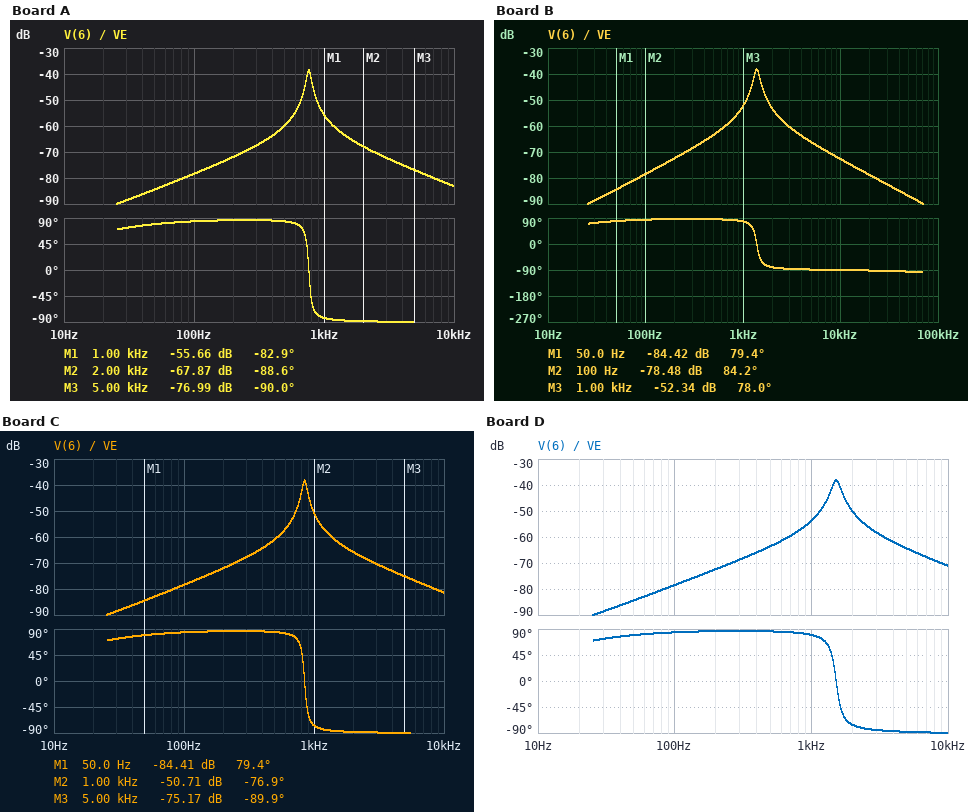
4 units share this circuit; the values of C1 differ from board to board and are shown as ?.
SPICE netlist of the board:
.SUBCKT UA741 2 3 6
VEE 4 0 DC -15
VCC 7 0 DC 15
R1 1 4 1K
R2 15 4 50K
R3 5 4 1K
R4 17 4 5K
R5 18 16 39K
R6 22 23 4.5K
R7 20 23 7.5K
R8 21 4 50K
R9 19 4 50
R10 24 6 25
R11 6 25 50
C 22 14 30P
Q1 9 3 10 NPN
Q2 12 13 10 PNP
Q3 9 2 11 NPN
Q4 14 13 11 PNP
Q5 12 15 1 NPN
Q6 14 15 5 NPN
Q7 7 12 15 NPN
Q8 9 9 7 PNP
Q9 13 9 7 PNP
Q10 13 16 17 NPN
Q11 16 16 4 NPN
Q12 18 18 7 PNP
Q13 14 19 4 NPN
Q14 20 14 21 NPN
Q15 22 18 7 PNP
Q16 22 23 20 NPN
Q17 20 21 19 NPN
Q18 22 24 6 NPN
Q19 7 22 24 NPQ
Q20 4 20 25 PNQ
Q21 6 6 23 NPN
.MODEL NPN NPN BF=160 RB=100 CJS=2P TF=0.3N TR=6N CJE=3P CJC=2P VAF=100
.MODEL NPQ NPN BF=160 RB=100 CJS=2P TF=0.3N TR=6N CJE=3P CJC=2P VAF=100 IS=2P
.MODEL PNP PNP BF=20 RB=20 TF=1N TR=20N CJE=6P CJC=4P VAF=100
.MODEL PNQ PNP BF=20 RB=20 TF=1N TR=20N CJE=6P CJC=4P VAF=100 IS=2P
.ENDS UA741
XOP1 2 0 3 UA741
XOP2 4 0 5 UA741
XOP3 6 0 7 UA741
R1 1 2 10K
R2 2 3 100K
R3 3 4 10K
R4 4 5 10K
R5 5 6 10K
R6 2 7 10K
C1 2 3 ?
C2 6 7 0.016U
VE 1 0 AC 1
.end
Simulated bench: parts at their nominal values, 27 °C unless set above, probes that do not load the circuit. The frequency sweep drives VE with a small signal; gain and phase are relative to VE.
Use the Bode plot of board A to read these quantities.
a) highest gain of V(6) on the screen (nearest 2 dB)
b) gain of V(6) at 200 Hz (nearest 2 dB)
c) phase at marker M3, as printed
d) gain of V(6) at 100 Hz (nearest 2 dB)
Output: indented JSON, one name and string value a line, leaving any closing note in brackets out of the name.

{
  "highest gain of V(6) on the screen": "-38 dB",
  "gain of V(6) at 200 Hz": "-72 dB",
  "phase at marker M3, as printed": "-90.0 deg",
  "gain of V(6) at 100 Hz": "-78 dB"
}
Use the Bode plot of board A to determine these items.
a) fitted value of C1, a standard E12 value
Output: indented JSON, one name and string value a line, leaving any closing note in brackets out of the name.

{
  "fitted value of C1, a standard E12 value": "27 nF"
}
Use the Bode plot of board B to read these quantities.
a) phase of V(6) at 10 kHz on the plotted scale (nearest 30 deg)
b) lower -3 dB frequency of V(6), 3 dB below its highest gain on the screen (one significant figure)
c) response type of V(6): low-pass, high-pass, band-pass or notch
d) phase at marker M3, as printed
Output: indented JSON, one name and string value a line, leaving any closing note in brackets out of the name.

{
  "phase of V(6) at 10 kHz on the plotted scale": "-90 deg",
  "lower -3 dB frequency of V(6), 3 dB below its highest gain on the screen": "1 kHz",
  "response type of V(6): low-pass, high-pass, band-pass or notch": "band-pass",
  "phase at marker M3, as printed": "78.0 deg"
}
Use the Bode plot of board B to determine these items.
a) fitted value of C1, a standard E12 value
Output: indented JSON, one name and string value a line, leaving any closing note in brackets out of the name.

{
  "fitted value of C1, a standard E12 value": "8.2 nF"
}
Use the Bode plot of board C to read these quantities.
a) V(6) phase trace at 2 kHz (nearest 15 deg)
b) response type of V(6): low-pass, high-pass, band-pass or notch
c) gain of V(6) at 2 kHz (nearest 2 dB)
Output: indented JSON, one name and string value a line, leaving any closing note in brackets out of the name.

{
  "V(6) phase trace at 2 kHz": "-90 deg",
  "response type of V(6): low-pass, high-pass, band-pass or notch": "band-pass",
  "gain of V(6) at 2 kHz": "-66 dB"
}
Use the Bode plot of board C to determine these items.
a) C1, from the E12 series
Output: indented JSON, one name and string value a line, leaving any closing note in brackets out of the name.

{
  "C1, from the E12 series": "22 nF"
}
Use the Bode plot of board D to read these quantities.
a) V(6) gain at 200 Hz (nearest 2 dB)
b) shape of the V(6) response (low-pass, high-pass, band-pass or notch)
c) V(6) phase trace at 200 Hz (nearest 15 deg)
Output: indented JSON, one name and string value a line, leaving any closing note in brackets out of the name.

{
  "V(6) gain at 200 Hz": "-72 dB",
  "shape of the V(6) response": "band-pass",
  "V(6) phase trace at 200 Hz": "90 deg"
}
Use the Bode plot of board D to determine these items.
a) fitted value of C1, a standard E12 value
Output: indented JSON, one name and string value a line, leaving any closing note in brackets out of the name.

{
  "fitted value of C1, a standard E12 value": "6.8 nF"
}
